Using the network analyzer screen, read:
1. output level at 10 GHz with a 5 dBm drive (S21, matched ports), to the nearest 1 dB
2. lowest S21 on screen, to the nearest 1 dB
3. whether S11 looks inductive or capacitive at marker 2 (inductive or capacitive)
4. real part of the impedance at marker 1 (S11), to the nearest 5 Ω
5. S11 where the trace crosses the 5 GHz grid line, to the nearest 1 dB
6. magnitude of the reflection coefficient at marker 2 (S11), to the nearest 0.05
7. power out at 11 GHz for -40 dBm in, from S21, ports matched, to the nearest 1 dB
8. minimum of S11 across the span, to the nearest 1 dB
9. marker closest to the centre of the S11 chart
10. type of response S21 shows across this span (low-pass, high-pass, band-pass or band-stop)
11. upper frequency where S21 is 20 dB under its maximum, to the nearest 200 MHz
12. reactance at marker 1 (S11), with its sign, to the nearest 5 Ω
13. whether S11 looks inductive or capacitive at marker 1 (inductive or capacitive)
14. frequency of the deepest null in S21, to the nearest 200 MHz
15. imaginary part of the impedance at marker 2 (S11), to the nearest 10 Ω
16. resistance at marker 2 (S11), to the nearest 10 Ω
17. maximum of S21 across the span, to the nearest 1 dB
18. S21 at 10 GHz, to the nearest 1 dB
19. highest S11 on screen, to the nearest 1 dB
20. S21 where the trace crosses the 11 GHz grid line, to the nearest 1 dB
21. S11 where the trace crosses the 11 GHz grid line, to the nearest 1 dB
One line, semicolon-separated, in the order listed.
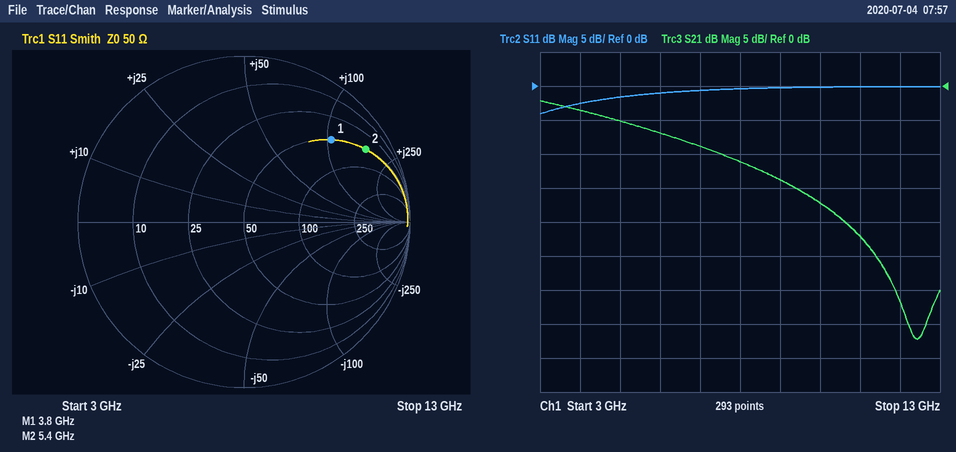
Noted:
-12 dBm; -37 dB; inductive; 50 Ω; -2 dB; 0.85; -62 dBm; -4 dB; marker 1; low-pass; 11.0 GHz; +105 Ω; inductive; 12.4 GHz; +170 Ω; 50 Ω; -2 dB; -17 dB; 0 dB; -22 dB; 0 dB
